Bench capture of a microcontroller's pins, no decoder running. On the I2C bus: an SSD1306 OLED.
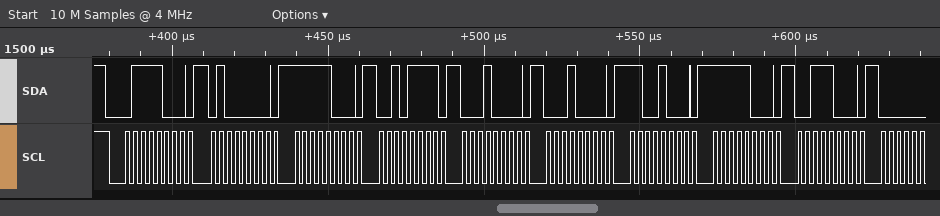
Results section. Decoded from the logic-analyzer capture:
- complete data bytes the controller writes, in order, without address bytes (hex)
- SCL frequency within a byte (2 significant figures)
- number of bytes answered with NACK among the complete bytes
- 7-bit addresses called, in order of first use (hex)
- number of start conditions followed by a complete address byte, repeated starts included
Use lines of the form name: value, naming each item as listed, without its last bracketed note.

complete data bytes the controller writes, in order, without address bytes: 40 F8 2F 10 10 C8 F8 38
SCL frequency within a byte: 400 kHz
number of bytes answered with NACK among the complete bytes: 0
7-bit addresses called, in order of first use: 0x3C
number of start conditions followed by a complete address byte, repeated starts included: 1
